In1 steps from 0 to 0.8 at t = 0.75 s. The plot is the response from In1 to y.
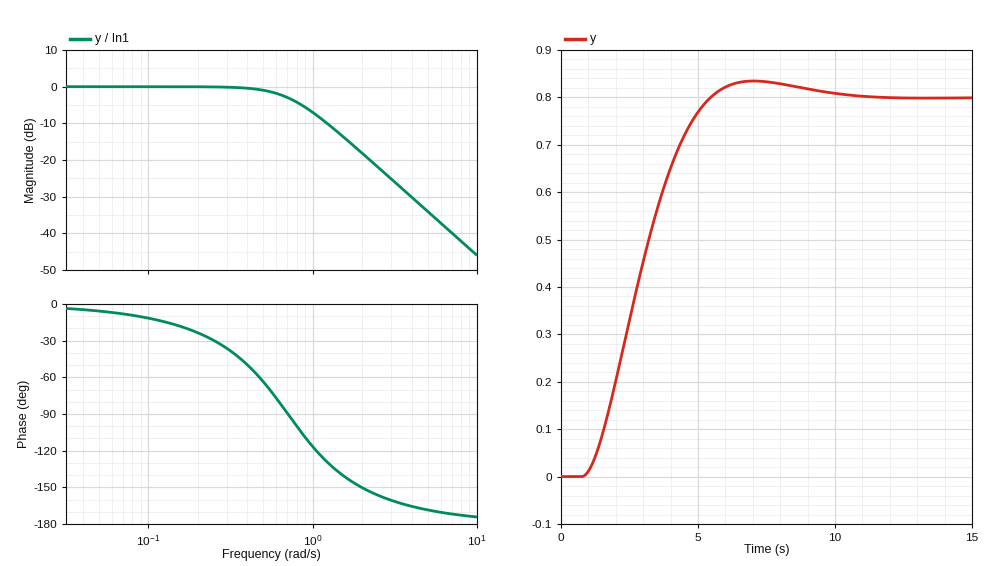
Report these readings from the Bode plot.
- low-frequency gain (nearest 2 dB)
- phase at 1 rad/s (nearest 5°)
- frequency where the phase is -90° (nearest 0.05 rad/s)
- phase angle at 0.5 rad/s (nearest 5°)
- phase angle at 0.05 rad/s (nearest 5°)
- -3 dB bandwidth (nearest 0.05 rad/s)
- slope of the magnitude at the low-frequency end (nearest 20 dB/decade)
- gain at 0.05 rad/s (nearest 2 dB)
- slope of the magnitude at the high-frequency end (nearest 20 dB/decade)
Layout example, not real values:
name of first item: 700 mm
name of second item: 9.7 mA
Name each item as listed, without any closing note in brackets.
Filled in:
low-frequency gain: 0 dB
phase at 1 rad/s: -115°
frequency where the phase is -90°: 0.70 rad/s
phase angle at 0.5 rad/s: -65°
phase angle at 0.05 rad/s: -5°
-3 dB bandwidth: 0.70 rad/s
slope of the magnitude at the low-frequency end: 0 dB/decade
gain at 0.05 rad/s: 0 dB
slope of the magnitude at the high-frequency end: -40 dB/decade
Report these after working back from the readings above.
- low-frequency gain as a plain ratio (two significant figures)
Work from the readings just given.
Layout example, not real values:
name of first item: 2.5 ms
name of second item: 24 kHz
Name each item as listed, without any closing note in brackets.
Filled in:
low-frequency gain as a plain ratio: 1.0
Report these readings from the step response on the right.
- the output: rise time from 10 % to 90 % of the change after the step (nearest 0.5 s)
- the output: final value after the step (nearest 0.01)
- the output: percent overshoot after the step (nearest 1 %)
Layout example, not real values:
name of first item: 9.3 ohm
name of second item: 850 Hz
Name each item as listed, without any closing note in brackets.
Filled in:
the output: rise time from 10 % to 90 % of the change after the step: 3.0 s
the output: final value after the step: 0.80
the output: percent overshoot after the step: 4 %
